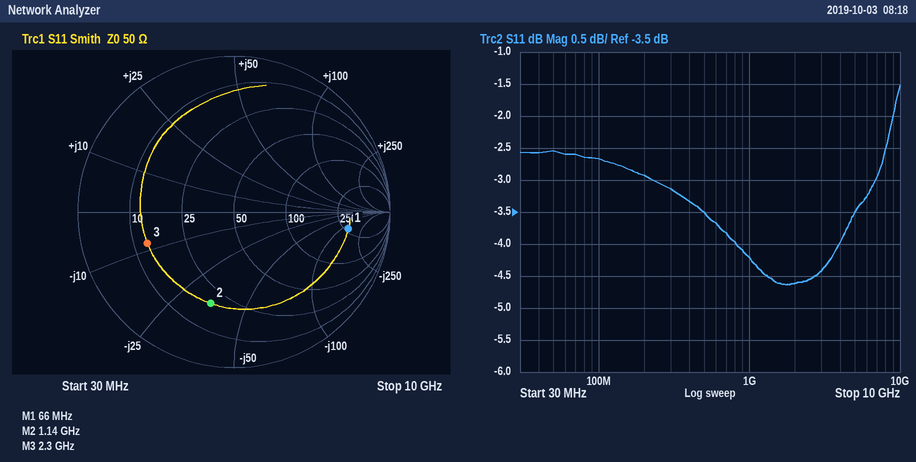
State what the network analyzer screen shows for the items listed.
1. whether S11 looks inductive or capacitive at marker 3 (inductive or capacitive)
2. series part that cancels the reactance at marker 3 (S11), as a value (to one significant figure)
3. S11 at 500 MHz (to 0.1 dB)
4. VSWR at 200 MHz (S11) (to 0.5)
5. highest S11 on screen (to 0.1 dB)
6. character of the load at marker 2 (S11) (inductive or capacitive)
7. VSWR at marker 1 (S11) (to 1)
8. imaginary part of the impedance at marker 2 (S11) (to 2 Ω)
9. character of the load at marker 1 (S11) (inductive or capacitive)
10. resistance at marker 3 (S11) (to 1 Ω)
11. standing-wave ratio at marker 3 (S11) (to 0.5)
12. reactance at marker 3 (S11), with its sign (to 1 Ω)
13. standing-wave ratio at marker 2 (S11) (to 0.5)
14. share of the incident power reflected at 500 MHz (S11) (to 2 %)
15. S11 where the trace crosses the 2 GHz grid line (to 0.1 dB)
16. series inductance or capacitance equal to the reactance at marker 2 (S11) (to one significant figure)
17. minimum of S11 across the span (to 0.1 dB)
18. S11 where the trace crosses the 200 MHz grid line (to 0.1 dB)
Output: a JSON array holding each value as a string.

["capacitive", "600 pH", "-3.5 dB", "6.0", "-1.5 dB", "capacitive", "7", "-36 Ω", "capacitive", "13 Ω", "4.0", "-8 Ω", "4.0", "44 %", "-4.6 dB", "4 pF", "-4.6 dB", "-2.9 dB"]
